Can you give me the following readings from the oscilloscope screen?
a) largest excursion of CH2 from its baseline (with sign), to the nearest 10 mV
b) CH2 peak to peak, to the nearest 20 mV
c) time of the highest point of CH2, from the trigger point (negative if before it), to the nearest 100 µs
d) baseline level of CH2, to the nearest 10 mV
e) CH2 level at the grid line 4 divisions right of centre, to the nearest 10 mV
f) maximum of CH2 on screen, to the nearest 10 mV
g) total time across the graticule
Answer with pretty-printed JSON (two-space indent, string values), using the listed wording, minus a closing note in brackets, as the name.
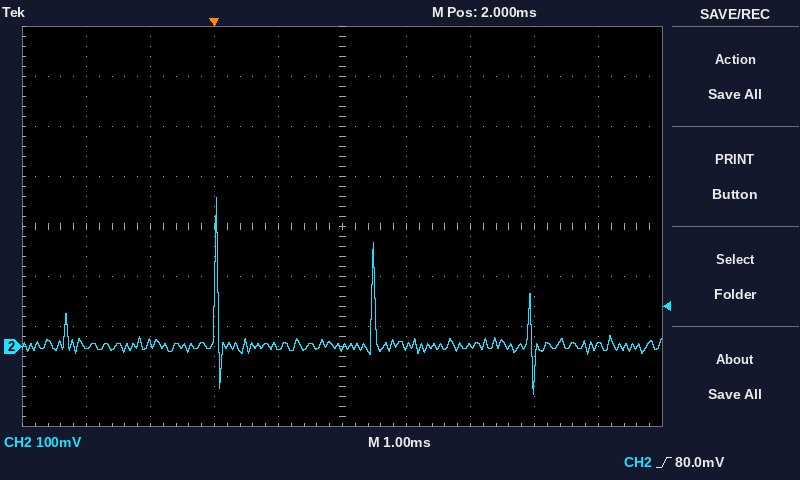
{
  "largest excursion of CH2 from its baseline (with sign), to the nearest 10 mV": "+300 mV",
  "CH2 peak to peak, to the nearest 20 mV": "400 mV",
  "time of the highest point of CH2, from the trigger point (negative if before it), to the nearest 100 µs": "0.0 ms",
  "baseline level of CH2, to the nearest 10 mV": "0 mV",
  "CH2 level at the grid line 4 divisions right of centre, to the nearest 10 mV": "0 mV",
  "maximum of CH2 on screen, to the nearest 10 mV": "300 mV",
  "total time across the graticule": "10 ms"
}
